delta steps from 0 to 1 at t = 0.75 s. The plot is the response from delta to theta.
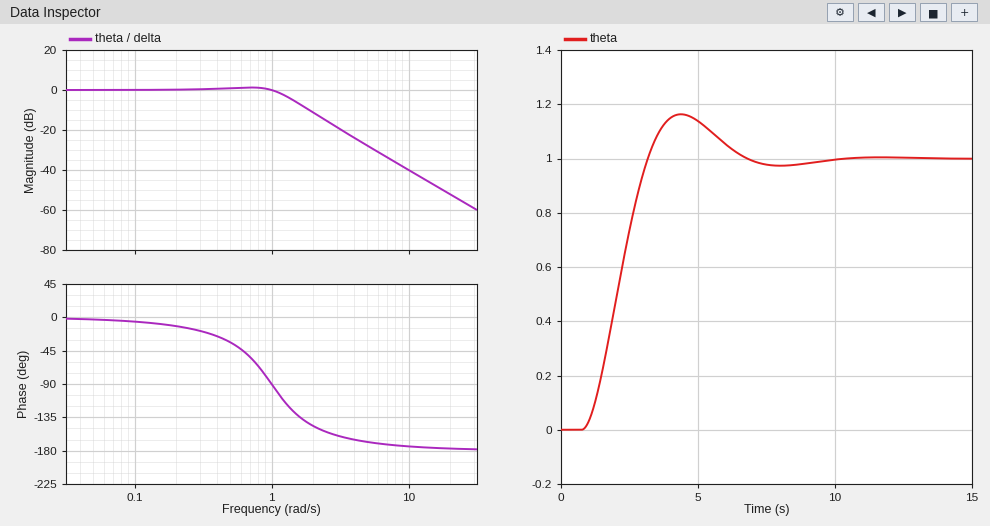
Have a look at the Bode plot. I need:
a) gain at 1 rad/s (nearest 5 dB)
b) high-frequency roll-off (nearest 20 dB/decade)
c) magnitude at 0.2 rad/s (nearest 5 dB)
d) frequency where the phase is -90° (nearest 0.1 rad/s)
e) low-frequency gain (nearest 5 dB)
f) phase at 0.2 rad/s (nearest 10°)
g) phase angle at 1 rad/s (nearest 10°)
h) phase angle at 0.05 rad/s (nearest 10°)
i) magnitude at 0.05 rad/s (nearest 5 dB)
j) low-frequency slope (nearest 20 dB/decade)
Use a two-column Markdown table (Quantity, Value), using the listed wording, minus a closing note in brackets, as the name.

| Quantity | Value |
|---|---|
| gain at 1 rad/s | 0 dB |
| high-frequency roll-off | -40 dB/decade |
| magnitude at 0.2 rad/s | 0 dB |
| frequency where the phase is -90° | 1.0 rad/s |
| low-frequency gain | 0 dB |
| phase at 0.2 rad/s | -10° |
| phase angle at 1 rad/s | -90° |
| phase angle at 0.05 rad/s | 0° |
| magnitude at 0.05 rad/s | 0 dB |
| low-frequency slope | 0 dB/decade |
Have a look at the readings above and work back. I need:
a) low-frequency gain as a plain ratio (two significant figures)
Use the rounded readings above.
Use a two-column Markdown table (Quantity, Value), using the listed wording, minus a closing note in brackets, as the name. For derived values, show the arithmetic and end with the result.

| Quantity | Value |
|---|---|
| low-frequency gain as a plain ratio | 10^(0 / 20) = 1.0 |
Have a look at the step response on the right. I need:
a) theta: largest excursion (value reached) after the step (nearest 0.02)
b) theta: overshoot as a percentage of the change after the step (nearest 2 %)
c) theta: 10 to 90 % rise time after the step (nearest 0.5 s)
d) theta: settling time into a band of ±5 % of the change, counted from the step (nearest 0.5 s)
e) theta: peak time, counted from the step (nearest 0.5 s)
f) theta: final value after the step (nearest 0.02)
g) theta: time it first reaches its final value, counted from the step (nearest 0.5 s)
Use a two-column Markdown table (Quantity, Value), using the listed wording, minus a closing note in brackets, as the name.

| Quantity | Value |
|---|---|
| theta: largest excursion (value reached) after the step | 1.16 |
| theta: overshoot as a percentage of the change after the step | 16 % |
| theta: 10 to 90 % rise time after the step | 1.5 s |
| theta: settling time into a band of ±5 % of the change, counted from the step | 5.5 s |
| theta: peak time, counted from the step | 3.5 s |
| theta: final value after the step | 1.00 |
| theta: time it first reaches its final value, counted from the step | 2.5 s |
